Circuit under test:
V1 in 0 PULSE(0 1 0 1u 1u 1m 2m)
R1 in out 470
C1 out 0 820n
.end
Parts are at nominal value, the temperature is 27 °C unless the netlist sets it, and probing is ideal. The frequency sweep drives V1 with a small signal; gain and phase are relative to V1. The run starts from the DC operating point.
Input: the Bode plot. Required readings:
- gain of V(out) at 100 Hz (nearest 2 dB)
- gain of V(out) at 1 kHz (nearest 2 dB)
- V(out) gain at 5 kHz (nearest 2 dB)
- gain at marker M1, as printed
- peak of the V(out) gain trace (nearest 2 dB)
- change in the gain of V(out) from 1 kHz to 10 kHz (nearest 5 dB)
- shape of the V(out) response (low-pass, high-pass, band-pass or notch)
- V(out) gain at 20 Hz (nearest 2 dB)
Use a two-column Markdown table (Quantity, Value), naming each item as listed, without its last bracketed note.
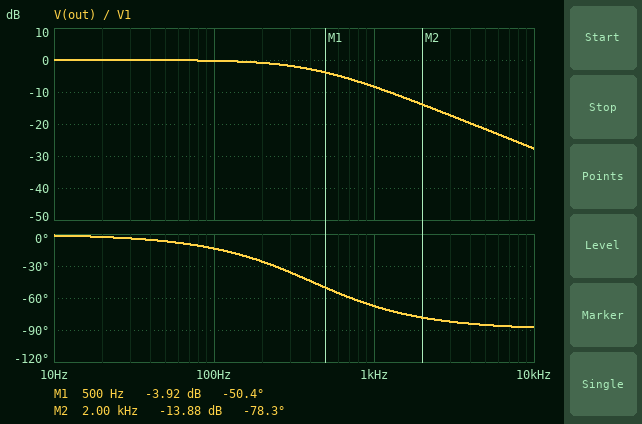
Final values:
| Quantity | Value |
|---|---|
| gain of V(out) at 100 Hz | 0 dB |
| gain of V(out) at 1 kHz | -8 dB |
| V(out) gain at 5 kHz | -22 dB |
| gain at marker M1, as printed | -3.92 dB |
| peak of the V(out) gain trace | 0 dB |
| change in the gain of V(out) from 1 kHz to 10 kHz | -20 dB |
| shape of the V(out) response | low-pass |
| V(out) gain at 20 Hz | 0 dB |
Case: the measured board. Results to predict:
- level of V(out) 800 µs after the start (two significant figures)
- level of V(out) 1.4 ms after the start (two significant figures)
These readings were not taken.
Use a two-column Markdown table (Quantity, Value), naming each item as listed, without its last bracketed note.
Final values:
| Quantity | Value |
|---|---|
| level of V(out) 800 µs after the start | 870 mV |
| level of V(out) 1.4 ms after the start | 330 mV |
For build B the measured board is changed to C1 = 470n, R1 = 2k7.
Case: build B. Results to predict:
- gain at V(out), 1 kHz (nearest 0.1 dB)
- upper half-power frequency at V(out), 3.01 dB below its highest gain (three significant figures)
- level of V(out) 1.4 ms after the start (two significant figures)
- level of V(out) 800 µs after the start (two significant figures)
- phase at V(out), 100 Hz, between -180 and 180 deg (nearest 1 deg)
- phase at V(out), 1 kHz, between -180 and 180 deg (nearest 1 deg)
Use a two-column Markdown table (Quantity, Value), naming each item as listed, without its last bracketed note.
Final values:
| Quantity | Value |
|---|---|
| gain at V(out), 1 kHz | -18.1 dB |
| upper half-power frequency at V(out), 3.01 dB below its highest gain | 125 Hz |
| level of V(out) 1.4 ms after the start | 400 mV |
| level of V(out) 800 µs after the start | 470 mV |
| phase at V(out), 100 Hz, between -180 and 180 deg | -39 deg |
| phase at V(out), 1 kHz, between -180 and 180 deg | -83 deg |
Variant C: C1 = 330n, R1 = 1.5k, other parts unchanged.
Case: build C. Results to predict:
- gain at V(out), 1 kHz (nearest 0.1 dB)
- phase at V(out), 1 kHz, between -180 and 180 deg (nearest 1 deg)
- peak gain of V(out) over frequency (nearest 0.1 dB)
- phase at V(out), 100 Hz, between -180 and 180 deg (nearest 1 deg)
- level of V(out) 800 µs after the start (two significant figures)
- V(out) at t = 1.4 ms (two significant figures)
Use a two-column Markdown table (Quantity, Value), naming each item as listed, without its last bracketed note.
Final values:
| Quantity | Value |
|---|---|
| gain at V(out), 1 kHz | -10.3 dB |
| phase at V(out), 1 kHz, between -180 and 180 deg | -72 deg |
| peak gain of V(out) over frequency | 0 dB |
| phase at V(out), 100 Hz, between -180 and 180 deg | -17 deg |
| level of V(out) 800 µs after the start | 800 mV |
| V(out) at t = 1.4 ms | 390 mV |
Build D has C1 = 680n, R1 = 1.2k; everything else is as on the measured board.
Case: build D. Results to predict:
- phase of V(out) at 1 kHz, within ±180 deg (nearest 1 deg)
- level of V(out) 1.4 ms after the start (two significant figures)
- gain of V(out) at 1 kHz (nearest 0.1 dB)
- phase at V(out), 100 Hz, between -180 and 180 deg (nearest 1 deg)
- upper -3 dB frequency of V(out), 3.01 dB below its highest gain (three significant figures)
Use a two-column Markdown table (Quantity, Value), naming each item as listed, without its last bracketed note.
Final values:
| Quantity | Value |
|---|---|
| phase of V(out) at 1 kHz, within ±180 deg | -79 deg |
| level of V(out) 1.4 ms after the start | 430 mV |
| gain of V(out) at 1 kHz | -14.4 dB |
| phase at V(out), 100 Hz, between -180 and 180 deg | -27 deg |
| upper -3 dB frequency of V(out), 3.01 dB below its highest gain | 195 Hz |
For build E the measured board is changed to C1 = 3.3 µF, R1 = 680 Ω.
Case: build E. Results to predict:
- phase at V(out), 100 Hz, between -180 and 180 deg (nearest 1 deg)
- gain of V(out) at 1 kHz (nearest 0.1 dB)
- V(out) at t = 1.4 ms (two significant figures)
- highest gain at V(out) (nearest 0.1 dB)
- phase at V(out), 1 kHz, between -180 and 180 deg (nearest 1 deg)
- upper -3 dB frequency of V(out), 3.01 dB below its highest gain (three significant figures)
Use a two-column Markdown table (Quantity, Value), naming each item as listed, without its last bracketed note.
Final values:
| Quantity | Value |
|---|---|
| phase at V(out), 100 Hz, between -180 and 180 deg | -55 deg |
| gain of V(out) at 1 kHz | -23.0 dB |
| V(out) at t = 1.4 ms | 300 mV |
| highest gain at V(out) | 0 dB |
| phase at V(out), 1 kHz, between -180 and 180 deg | -86 deg |
| upper -3 dB frequency of V(out), 3.01 dB below its highest gain | 70.9 Hz |
